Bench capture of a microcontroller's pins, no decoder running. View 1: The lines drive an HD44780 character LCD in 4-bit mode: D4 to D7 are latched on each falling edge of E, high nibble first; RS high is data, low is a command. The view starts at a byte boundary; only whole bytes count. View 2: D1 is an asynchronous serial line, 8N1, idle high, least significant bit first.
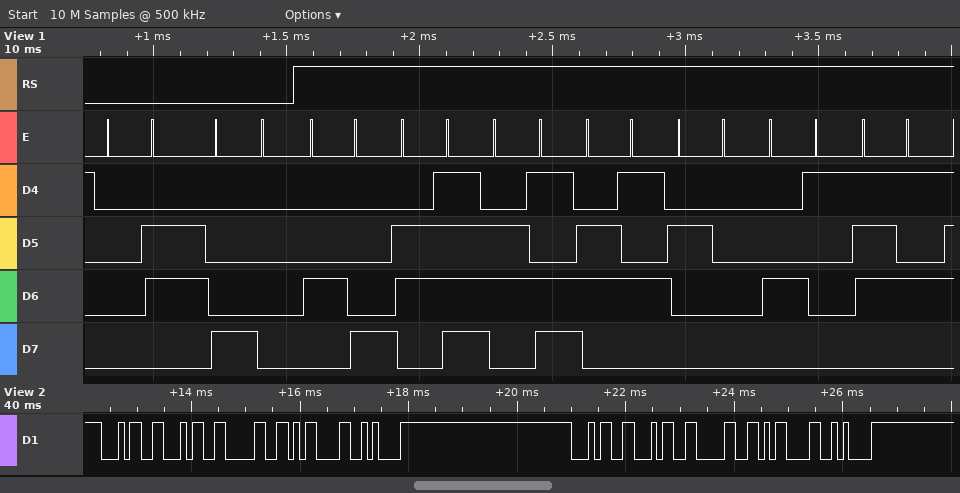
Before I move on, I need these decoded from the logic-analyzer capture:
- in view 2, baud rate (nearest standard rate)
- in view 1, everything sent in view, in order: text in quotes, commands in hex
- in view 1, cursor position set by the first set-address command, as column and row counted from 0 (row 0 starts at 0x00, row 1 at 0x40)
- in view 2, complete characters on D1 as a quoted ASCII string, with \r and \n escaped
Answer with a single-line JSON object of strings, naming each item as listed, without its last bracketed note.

{"in view 2, baud rate": "9600 baud", "in view 1, everything sent in view, in order: text in quotes, commands in hex": "0x06 0x80 \"Home Au\"", "in view 1, cursor position set by the first set-address command, as column and row counted from 0": "column 0, row 0", "in view 2, complete characters on D1 as a quoted ASCII string, with \\r and \\n escaped": "\"440\\r\\n440\\r\\n\""}
